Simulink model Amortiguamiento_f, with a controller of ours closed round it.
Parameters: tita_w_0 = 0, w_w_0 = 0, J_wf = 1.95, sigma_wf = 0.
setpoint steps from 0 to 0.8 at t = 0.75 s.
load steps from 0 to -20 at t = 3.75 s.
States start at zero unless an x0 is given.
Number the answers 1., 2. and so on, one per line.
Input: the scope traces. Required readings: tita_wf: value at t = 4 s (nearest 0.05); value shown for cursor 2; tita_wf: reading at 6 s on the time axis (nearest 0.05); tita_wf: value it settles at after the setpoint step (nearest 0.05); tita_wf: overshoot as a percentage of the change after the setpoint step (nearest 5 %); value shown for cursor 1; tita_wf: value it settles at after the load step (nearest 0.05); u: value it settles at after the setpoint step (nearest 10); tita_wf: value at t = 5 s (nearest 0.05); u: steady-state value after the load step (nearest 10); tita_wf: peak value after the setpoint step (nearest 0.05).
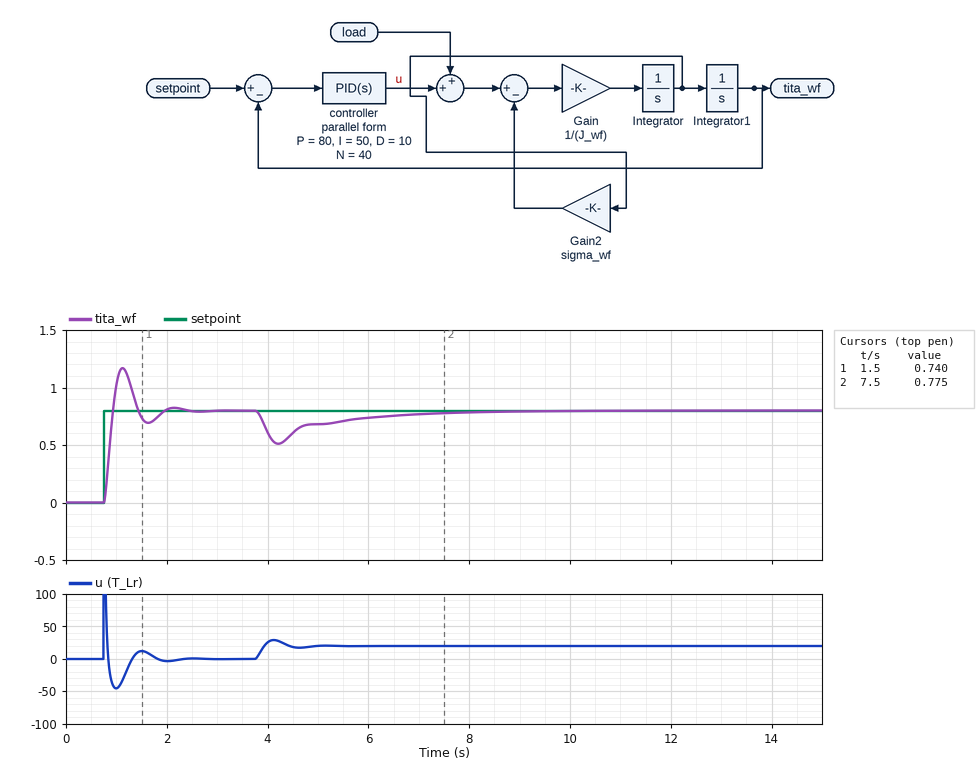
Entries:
1. 0.60
2. 0.775
3. 0.75
4. 0.80
5. 45 %
6. 0.740
7. 0.80
8. 0
9. 0.70
10. 20
11. 1.15
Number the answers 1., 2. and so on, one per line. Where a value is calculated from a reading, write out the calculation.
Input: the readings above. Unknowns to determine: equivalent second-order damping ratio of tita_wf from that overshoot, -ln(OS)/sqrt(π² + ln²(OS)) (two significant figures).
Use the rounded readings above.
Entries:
1. ln(0.45) = -0.799; 0.799 / sqrt(9.870 + 0.638) = 0.25
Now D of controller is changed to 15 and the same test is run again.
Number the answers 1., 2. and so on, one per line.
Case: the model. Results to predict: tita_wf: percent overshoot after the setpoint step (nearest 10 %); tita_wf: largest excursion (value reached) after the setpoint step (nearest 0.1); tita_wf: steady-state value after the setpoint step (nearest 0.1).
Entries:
1. 30 %
2. 1.1
3. 0.8
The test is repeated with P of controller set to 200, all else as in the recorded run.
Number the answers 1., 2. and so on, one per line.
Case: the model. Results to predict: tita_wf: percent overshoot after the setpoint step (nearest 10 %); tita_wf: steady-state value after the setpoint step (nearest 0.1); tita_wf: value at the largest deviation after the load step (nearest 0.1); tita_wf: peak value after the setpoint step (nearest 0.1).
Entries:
1. 60 %
2. 0.8
3. 0.7
4. 1.3
